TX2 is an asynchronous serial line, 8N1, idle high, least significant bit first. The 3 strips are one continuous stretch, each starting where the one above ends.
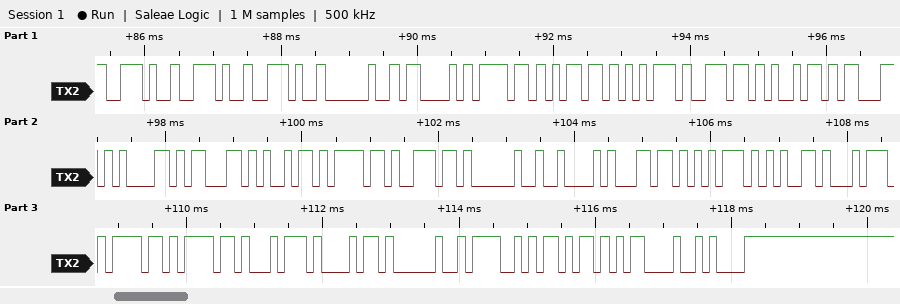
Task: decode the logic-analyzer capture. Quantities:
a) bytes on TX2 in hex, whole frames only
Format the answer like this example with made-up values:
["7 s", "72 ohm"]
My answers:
["2E 2E 2E 20 43 6F 6D 75 6E 69 63 61 63 69 6F 6E 20 42 6C 75 65 74 6F 6F 74 68 20 4F 6B 0D 0A"]
